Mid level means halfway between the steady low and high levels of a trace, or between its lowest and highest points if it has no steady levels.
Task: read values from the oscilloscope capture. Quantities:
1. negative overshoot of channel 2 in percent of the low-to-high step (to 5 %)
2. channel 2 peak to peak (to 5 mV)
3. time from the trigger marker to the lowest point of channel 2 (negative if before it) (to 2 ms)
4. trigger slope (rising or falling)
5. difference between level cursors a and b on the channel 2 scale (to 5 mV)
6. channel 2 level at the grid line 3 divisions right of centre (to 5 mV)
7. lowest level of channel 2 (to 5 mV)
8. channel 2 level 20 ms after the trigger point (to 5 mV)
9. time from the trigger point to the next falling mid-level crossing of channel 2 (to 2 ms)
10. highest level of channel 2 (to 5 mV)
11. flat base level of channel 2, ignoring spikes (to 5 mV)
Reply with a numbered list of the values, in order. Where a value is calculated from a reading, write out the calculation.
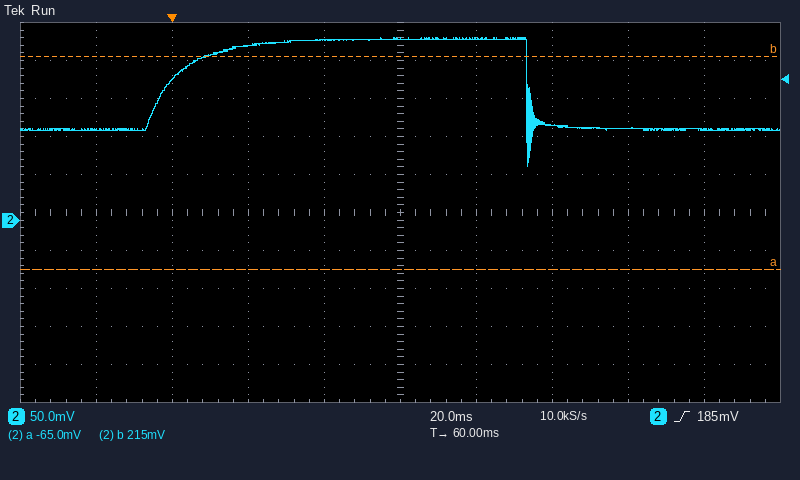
1. 40 %
2. 240 mV − (70 mV) = 170 mV
3. +94 ms
4. rising
5. 280 mV
6. 120 mV
7. 70 mV
8. 230 mV
9. 94 ms
10. 240 mV
11. 120 mV
